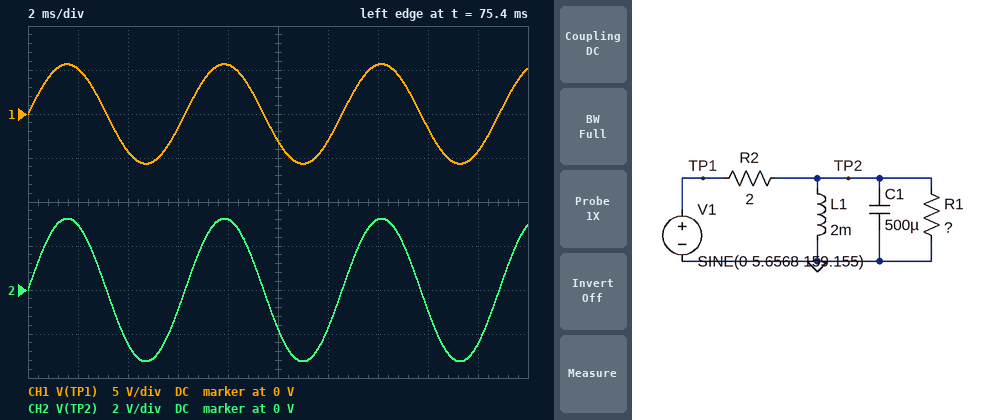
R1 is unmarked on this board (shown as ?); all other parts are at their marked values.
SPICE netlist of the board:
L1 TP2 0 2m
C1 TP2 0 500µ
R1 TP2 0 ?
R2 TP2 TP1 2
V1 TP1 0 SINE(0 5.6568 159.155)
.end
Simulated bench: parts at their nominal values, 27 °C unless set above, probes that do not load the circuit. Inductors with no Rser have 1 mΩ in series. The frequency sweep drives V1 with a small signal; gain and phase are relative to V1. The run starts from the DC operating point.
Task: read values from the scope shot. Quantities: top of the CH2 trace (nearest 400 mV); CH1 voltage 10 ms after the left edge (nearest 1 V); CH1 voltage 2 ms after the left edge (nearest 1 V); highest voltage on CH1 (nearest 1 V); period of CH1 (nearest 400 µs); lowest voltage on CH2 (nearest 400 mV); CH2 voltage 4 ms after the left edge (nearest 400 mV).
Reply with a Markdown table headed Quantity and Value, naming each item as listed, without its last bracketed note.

| Quantity | Value |
|---|---|
| top of the CH2 trace | 3.2 V |
| CH1 voltage 10 ms after the left edge | -3 V |
| CH1 voltage 2 ms after the left edge | 5 V |
| highest voltage on CH1 | 6 V |
| period of CH1 | 6.4 ms |
| lowest voltage on CH2 | -3.2 V |
| CH2 voltage 4 ms after the left edge | -2.4 V |
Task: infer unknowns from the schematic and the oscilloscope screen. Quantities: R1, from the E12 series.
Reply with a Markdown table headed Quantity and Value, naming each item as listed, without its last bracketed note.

| Quantity | Value |
|---|---|
| R1, from the E12 series | 2.7 Ω |
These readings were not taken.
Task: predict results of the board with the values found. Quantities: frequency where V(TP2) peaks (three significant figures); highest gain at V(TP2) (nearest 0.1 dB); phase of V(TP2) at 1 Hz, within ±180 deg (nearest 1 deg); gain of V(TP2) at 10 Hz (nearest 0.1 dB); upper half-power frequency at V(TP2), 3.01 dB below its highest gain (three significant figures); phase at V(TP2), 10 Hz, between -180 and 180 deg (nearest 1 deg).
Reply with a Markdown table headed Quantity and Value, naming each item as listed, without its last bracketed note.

| Quantity | Value |
|---|---|
| frequency where V(TP2) peaks | 159 Hz |
| highest gain at V(TP2) | -4.8 dB |
| phase of V(TP2) at 1 Hz, within ±180 deg | 85 deg |
| gain of V(TP2) at 10 Hz | -24.1 dB |
| upper half-power frequency at V(TP2), 3.01 dB below its highest gain | 350 Hz |
| phase at V(TP2), 10 Hz, between -180 and 180 deg | 83 deg |
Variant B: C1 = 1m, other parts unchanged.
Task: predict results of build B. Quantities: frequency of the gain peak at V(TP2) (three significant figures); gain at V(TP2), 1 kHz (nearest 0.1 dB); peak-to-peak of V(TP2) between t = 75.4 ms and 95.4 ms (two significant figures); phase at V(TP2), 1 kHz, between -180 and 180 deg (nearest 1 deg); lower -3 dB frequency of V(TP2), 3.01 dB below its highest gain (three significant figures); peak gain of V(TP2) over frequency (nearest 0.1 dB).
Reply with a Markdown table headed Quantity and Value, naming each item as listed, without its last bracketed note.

| Quantity | Value |
|---|---|
| frequency of the gain peak at V(TP2) | 113 Hz |
| gain at V(TP2), 1 kHz | -22.0 dB |
| peak-to-peak of V(TP2) between t = 75.4 ms and 95.4 ms | 5.6 V |
| phase at V(TP2), 1 kHz, between -180 and 180 deg | -82 deg |
| lower -3 dB frequency of V(TP2), 3.01 dB below its highest gain | 62.9 Hz |
| peak gain of V(TP2) over frequency | -4.8 dB |
